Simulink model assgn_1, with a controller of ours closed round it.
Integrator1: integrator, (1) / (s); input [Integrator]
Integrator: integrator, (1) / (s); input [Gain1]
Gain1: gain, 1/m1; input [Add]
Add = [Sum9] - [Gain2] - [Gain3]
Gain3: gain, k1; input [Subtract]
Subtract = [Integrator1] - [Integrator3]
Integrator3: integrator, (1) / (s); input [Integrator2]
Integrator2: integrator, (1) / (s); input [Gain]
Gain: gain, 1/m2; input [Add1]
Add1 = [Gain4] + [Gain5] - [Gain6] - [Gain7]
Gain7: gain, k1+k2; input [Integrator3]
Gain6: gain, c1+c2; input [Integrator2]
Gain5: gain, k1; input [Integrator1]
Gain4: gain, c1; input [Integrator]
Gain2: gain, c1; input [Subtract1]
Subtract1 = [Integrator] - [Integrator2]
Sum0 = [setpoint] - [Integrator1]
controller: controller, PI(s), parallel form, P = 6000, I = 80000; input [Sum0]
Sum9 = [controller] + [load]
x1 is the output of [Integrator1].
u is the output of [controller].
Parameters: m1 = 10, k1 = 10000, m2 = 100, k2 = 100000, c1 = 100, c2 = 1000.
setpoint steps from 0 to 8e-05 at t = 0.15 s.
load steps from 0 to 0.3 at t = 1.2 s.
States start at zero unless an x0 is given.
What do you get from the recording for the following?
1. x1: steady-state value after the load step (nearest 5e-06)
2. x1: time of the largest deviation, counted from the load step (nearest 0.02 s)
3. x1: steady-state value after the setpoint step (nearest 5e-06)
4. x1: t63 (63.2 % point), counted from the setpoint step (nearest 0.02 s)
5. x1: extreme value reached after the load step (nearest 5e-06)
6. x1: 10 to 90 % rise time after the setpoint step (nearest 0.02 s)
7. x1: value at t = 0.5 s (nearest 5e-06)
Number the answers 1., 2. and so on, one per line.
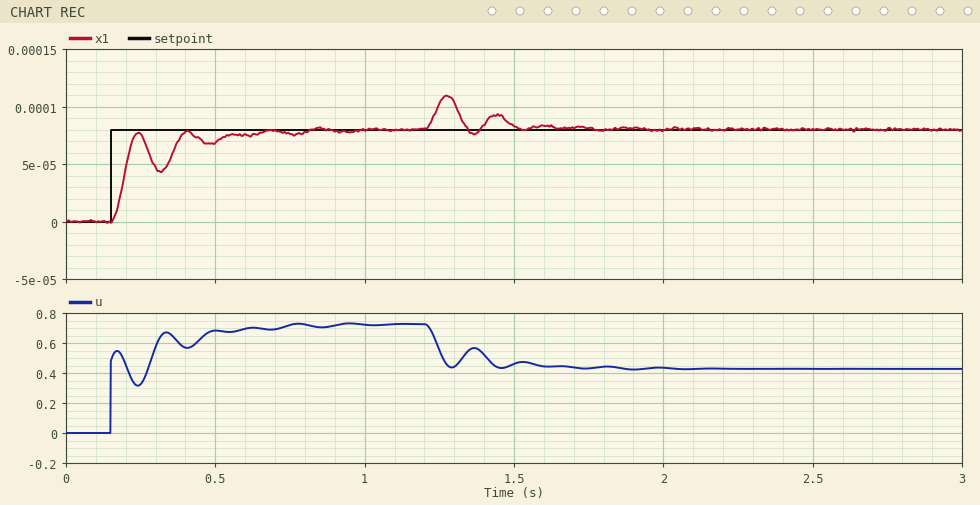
1. 0.000080
2. 0.08 s
3. 0.000080
4. 0.06 s
5. 0.000110
6. 0.06 s
7. 0.000070
